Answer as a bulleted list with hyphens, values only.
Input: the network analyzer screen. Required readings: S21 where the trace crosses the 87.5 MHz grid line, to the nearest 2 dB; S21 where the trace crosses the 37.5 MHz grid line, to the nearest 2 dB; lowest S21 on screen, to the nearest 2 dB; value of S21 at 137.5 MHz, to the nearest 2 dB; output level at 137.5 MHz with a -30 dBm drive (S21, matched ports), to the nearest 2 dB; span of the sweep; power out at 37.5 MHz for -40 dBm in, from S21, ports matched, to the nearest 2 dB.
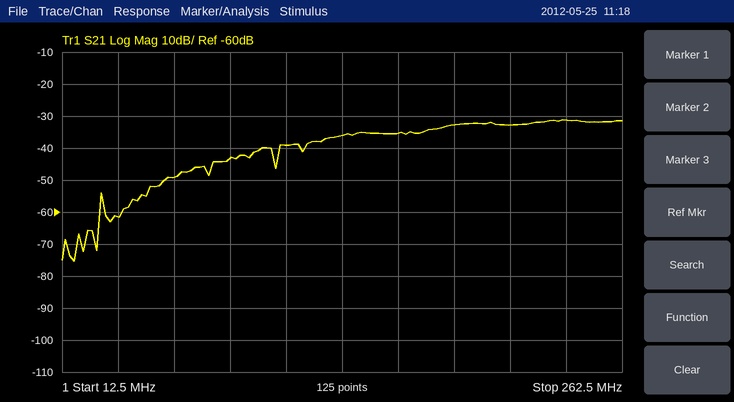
- -44 dB
- -62 dB
- -76 dB
- -36 dB
- -66 dBm
- 250 MHz
- -102 dBm
